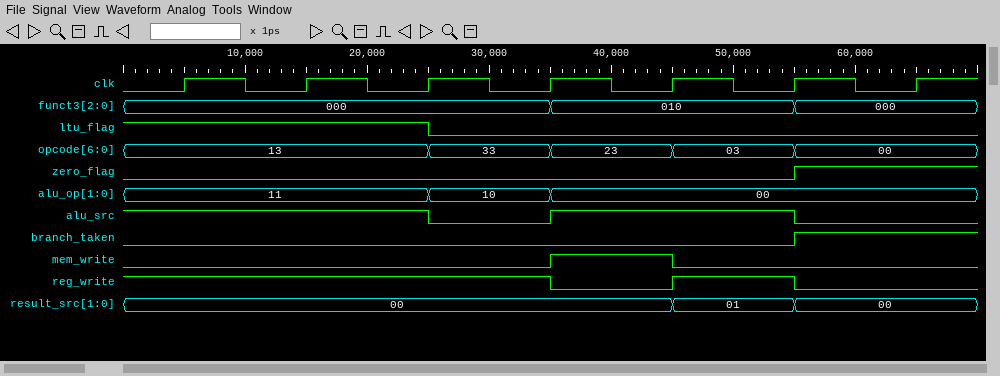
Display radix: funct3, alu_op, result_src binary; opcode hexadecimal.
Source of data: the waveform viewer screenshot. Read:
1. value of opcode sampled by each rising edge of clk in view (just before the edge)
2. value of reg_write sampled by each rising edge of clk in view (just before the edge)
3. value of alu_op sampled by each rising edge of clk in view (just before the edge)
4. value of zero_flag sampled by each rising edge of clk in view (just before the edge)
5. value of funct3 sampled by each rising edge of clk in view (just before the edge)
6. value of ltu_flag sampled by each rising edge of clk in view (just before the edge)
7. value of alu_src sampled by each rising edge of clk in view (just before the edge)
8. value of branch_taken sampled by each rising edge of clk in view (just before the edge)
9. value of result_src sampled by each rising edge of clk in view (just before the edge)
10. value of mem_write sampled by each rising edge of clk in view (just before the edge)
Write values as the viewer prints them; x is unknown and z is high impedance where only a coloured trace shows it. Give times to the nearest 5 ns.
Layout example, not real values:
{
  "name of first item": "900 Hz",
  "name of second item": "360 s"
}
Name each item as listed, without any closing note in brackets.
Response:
{
  "value of opcode sampled by each rising edge of clk in view": "13, 13, 13, 33, 23, 03, 00",
  "value of reg_write sampled by each rising edge of clk in view": "1 1 1 1 0 1 0",
  "value of alu_op sampled by each rising edge of clk in view": "11, 11, 11, 10, 00, 00, 00",
  "value of zero_flag sampled by each rising edge of clk in view": "0 0 0 0 0 0 1",
  "value of funct3 sampled by each rising edge of clk in view": "000, 000, 000, 000, 010, 010, 000",
  "value of ltu_flag sampled by each rising edge of clk in view": "1 1 1 0 0 0 0",
  "value of alu_src sampled by each rising edge of clk in view": "1 1 1 0 1 1 0",
  "value of branch_taken sampled by each rising edge of clk in view": "0 0 0 0 0 0 1",
  "value of result_src sampled by each rising edge of clk in view": "00, 00, 00, 00, 00, 01, 00",
  "value of mem_write sampled by each rising edge of clk in view": "0 0 0 0 1 0 0"
}
